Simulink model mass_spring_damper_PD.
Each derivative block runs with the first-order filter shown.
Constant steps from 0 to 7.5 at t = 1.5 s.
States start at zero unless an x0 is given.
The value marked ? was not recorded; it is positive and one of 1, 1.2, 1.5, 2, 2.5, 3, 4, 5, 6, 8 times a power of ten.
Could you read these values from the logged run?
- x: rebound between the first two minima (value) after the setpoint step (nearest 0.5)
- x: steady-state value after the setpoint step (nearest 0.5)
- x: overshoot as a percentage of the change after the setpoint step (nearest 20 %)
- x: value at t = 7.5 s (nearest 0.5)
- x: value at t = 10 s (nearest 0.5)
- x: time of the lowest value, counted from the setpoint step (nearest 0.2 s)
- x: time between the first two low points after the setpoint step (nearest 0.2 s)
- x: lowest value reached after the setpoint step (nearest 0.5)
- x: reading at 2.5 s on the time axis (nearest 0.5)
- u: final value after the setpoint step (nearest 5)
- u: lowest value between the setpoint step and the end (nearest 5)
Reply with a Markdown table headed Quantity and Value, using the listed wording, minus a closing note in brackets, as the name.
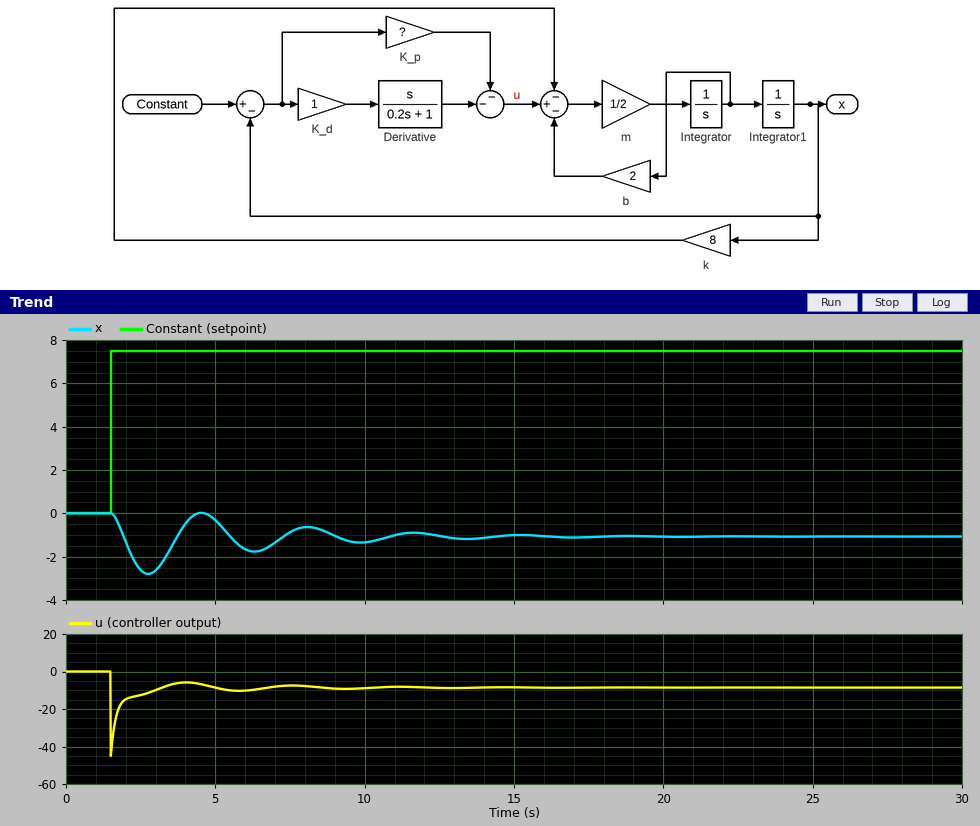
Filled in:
| Quantity | Value |
|---|---|
| x: rebound between the first two minima (value) after the setpoint step | 0.0 |
| x: steady-state value after the setpoint step | -1.0 |
| x: overshoot as a percentage of the change after the setpoint step | 160 % |
| x: value at t = 7.5 s | -1.0 |
| x: value at t = 10 s | -1.5 |
| x: time of the lowest value, counted from the setpoint step | 1.2 s |
| x: time between the first two low points after the setpoint step | 3.6 s |
| x: lowest value reached after the setpoint step | -3.0 |
| x: reading at 2.5 s on the time axis | -2.5 |
| u: final value after the setpoint step | -10 |
| u: lowest value between the setpoint step and the end | -45 |
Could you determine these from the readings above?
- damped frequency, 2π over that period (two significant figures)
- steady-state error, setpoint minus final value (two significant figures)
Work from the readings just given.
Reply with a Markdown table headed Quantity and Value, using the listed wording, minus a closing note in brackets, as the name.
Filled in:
| Quantity | Value |
|---|---|
| damped frequency, 2π over that period | 1.7 rad/s |
| steady-state error, setpoint minus final value | 8.5 |
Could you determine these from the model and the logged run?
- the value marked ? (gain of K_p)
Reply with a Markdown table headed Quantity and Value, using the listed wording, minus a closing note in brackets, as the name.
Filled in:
| Quantity | Value |
|---|---|
| the value marked ? | 1 |
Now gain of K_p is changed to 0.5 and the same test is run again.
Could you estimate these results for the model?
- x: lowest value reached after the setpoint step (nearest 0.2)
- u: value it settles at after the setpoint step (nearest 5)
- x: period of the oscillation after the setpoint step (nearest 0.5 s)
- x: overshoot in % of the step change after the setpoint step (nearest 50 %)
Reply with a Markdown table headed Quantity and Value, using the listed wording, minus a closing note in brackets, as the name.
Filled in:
| Quantity | Value |
|---|---|
| x: lowest value reached after the setpoint step | -2.0 |
| u: value it settles at after the setpoint step | -5 |
| x: period of the oscillation after the setpoint step | 3.5 s |
| x: overshoot in % of the step change after the setpoint step | 300 % |
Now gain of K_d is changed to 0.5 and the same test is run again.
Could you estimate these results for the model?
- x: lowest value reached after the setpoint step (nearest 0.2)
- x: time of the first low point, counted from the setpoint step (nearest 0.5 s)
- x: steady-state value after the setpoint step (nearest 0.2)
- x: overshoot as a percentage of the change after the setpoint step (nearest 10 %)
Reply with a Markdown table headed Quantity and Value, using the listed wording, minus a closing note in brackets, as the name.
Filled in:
| Quantity | Value |
|---|---|
| x: lowest value reached after the setpoint step | -2.0 |
| x: time of the first low point, counted from the setpoint step | 1.5 s |
| x: steady-state value after the setpoint step | -1.0 |
| x: overshoot as a percentage of the change after the setpoint step | 90 % |
